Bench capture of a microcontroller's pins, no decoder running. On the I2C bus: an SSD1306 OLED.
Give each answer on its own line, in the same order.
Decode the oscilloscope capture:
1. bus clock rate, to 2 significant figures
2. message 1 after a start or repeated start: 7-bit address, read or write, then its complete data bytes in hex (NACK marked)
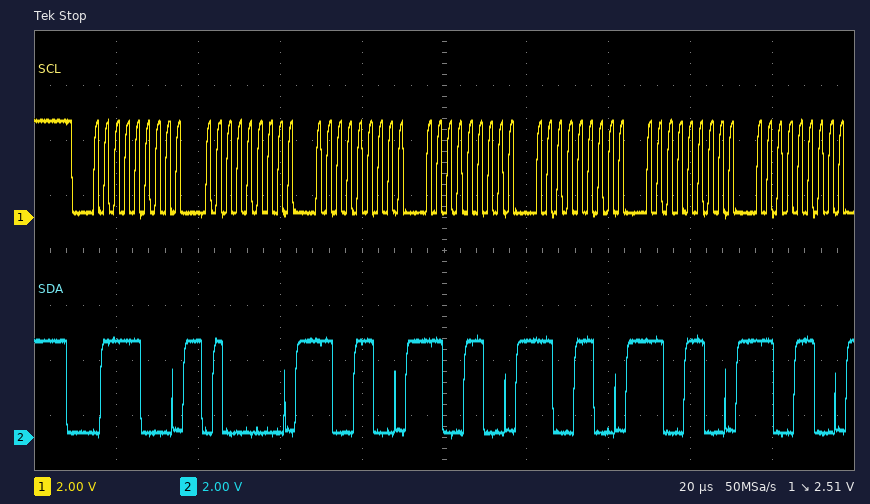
400 kHz
0x3C write: 40 CC CC CC CC CC
